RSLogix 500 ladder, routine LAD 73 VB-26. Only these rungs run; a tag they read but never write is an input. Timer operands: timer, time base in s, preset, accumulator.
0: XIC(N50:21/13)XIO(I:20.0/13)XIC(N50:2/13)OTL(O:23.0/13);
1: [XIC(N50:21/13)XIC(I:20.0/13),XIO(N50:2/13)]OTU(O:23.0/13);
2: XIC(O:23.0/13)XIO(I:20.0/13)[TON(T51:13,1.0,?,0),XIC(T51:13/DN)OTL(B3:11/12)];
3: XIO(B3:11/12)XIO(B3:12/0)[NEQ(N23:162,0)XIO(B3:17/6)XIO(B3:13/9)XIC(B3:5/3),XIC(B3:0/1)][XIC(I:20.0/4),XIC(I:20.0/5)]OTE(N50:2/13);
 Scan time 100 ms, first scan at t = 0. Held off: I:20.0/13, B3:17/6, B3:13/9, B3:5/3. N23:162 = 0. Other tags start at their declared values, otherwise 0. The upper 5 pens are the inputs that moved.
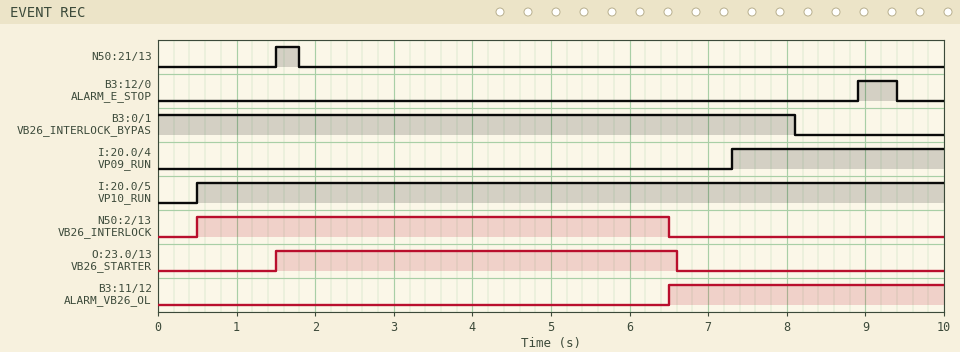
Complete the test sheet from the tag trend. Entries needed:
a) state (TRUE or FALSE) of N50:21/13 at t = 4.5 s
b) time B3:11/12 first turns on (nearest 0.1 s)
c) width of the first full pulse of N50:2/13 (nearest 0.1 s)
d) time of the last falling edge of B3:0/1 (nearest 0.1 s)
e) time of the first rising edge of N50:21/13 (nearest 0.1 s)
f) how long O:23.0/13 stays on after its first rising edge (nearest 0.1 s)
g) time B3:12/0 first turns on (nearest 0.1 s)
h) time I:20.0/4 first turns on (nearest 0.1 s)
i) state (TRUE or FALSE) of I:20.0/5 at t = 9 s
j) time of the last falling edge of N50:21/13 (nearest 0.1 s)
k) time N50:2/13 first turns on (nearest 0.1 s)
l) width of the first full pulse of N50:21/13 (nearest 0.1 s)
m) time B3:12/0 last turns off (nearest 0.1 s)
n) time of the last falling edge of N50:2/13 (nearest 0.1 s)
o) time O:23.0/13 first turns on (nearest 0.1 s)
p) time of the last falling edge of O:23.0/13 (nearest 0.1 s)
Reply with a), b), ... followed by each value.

a) FALSE
b) 6.5 s
c) 6.0 s
d) 8.1 s
e) 1.5 s
f) 5.1 s
g) 8.9 s
h) 7.3 s
i) TRUE
j) 1.8 s
k) 0.5 s
l) 0.3 s
m) 9.4 s
n) 6.5 s
o) 1.5 s
p) 6.6 s
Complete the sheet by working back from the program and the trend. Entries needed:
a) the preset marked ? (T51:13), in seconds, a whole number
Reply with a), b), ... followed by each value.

a) 5 s
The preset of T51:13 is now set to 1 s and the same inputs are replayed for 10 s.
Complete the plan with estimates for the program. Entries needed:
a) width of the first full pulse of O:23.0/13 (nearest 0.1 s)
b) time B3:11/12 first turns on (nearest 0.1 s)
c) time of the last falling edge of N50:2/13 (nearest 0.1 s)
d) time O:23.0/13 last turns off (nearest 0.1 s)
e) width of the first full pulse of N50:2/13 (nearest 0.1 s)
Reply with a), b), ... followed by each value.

a) 1.1 s
b) 2.5 s
c) 2.5 s
d) 2.6 s
e) 2.0 s
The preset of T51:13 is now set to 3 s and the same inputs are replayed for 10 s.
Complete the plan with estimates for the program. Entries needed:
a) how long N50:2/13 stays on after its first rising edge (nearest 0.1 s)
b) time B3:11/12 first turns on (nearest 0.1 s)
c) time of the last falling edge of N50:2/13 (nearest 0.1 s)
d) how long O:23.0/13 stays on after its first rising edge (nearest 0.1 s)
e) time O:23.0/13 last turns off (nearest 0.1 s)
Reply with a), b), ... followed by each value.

a) 4.0 s
b) 4.5 s
c) 4.5 s
d) 3.1 s
e) 4.6 s
